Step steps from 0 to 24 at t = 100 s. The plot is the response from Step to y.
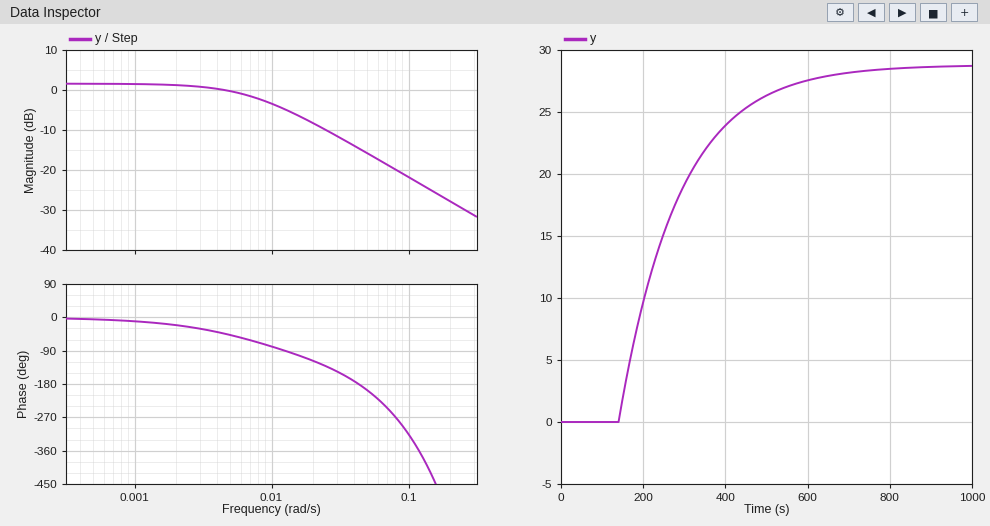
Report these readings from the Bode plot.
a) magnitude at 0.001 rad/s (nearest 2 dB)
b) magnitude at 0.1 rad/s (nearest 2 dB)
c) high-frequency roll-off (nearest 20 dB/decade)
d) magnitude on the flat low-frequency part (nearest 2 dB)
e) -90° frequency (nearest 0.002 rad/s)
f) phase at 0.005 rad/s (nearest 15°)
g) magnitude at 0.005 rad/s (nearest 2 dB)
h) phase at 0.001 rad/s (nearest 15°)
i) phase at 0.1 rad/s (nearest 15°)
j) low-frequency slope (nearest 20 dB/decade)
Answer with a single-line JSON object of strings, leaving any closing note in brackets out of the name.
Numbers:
{"magnitude at 0.001 rad/s": "2 dB", "magnitude at 0.1 rad/s": "-22 dB", "high-frequency roll-off": "-20 dB/decade", "magnitude on the flat low-frequency part": "2 dB", "-90° frequency": "0.012 rad/s", "phase at 0.005 rad/s": "-45°", "magnitude at 0.005 rad/s": "0 dB", "phase at 0.001 rad/s": "-15°", "phase at 0.1 rad/s": "-315°", "low-frequency slope": "0 dB/decade"}
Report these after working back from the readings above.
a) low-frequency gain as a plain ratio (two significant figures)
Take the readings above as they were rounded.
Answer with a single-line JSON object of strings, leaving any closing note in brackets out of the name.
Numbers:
{"low-frequency gain as a plain ratio": "1.3"}
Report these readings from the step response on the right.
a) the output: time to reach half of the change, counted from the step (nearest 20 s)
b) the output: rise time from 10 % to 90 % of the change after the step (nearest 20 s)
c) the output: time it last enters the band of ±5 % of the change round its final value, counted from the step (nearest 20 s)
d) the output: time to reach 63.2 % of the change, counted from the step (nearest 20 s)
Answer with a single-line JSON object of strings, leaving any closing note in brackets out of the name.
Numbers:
{"the output: time to reach half of the change, counted from the step": "140 s", "the output: rise time from 10 % to 90 % of the change after the step": "320 s", "the output: time it last enters the band of ±5 % of the change round its final value, counted from the step": "480 s", "the output: time to reach 63.2 % of the change, counted from the step": "180 s"}
